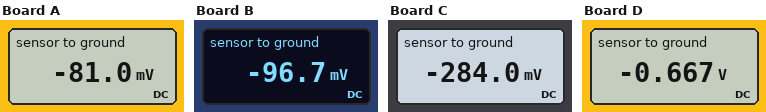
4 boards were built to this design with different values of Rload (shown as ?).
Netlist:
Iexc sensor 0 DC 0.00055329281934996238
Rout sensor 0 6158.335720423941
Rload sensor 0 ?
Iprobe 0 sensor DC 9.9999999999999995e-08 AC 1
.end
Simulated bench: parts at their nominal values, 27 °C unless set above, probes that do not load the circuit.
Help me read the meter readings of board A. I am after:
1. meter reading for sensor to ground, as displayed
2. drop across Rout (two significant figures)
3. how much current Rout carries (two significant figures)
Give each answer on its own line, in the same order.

-81.0 mV
81 mV
13 µA
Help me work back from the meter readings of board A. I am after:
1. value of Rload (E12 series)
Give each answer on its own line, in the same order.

150 Ω
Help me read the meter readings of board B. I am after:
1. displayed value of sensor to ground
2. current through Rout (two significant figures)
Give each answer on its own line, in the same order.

-96.7 mV
16 µA
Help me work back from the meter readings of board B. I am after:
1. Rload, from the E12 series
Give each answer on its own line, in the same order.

180 Ω
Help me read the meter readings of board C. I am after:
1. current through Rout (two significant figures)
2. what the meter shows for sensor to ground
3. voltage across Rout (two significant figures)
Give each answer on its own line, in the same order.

46 µA
-284.0 mV
280 mV
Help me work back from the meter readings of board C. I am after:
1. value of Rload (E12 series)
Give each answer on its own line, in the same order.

560 Ω
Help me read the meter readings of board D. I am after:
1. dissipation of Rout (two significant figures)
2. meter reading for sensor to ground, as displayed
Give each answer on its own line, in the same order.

72 µW
-0.667 V
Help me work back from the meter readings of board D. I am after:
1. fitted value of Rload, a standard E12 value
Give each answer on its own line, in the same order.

1.5 kΩ
